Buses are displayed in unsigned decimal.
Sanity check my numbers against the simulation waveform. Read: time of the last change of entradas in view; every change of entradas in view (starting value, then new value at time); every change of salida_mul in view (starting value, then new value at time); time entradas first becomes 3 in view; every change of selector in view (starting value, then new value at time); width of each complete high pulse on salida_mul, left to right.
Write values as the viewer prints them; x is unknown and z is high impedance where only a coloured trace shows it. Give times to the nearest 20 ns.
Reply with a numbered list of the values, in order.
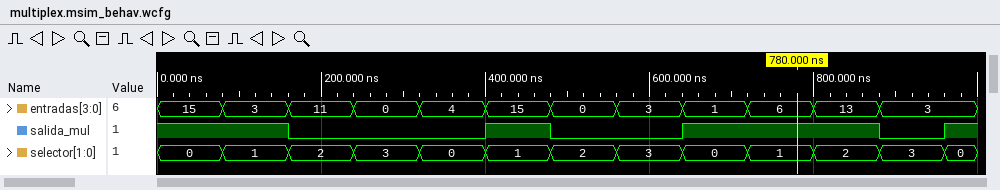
1. 880 ns
2. 15, 3 at 80 ns, 11 at 160 ns, 0 at 240 ns, 4 at 320 ns, 15 at 400 ns, 0 at 480 ns, 3 at 560 ns, 1 at 640 ns, 6 at 720 ns, 13 at 800 ns, 3 at 880 ns
3. 1, 0 at 160 ns, 1 at 400 ns, 0 at 480 ns, 1 at 640 ns, 0 at 880 ns, 1 at 960 ns
4. 80 ns
5. 0, 1 at 80 ns, 2 at 160 ns, 3 at 240 ns, 0 at 320 ns, 1 at 400 ns, 2 at 480 ns, 3 at 560 ns, 0 at 640 ns, 1 at 720 ns, 2 at 800 ns, 3 at 880 ns, 0 at 960 ns
6. 80 ns, 240 ns
